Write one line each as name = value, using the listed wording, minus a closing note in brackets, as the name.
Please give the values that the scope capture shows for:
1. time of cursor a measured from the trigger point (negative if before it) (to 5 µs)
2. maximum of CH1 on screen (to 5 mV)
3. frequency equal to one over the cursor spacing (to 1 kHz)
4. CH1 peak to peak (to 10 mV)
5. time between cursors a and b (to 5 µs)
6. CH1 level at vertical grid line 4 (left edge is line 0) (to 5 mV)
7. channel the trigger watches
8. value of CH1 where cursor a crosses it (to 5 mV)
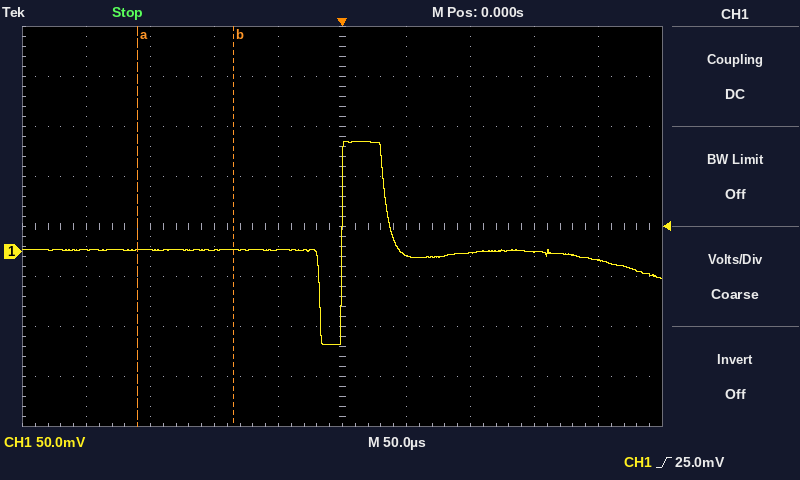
time of cursor a measured from the trigger point (negative if before it) = -160 µs
maximum of CH1 on screen = 110 mV
frequency equal to one over the cursor spacing = 13 kHz
CH1 peak to peak = 200 mV
time between cursors a and b = 75 µs
CH1 level at vertical grid line 4 (left edge is line 0) = 0 mV
channel the trigger watches = CH1
value of CH1 where cursor a crosses it = 0 mV
